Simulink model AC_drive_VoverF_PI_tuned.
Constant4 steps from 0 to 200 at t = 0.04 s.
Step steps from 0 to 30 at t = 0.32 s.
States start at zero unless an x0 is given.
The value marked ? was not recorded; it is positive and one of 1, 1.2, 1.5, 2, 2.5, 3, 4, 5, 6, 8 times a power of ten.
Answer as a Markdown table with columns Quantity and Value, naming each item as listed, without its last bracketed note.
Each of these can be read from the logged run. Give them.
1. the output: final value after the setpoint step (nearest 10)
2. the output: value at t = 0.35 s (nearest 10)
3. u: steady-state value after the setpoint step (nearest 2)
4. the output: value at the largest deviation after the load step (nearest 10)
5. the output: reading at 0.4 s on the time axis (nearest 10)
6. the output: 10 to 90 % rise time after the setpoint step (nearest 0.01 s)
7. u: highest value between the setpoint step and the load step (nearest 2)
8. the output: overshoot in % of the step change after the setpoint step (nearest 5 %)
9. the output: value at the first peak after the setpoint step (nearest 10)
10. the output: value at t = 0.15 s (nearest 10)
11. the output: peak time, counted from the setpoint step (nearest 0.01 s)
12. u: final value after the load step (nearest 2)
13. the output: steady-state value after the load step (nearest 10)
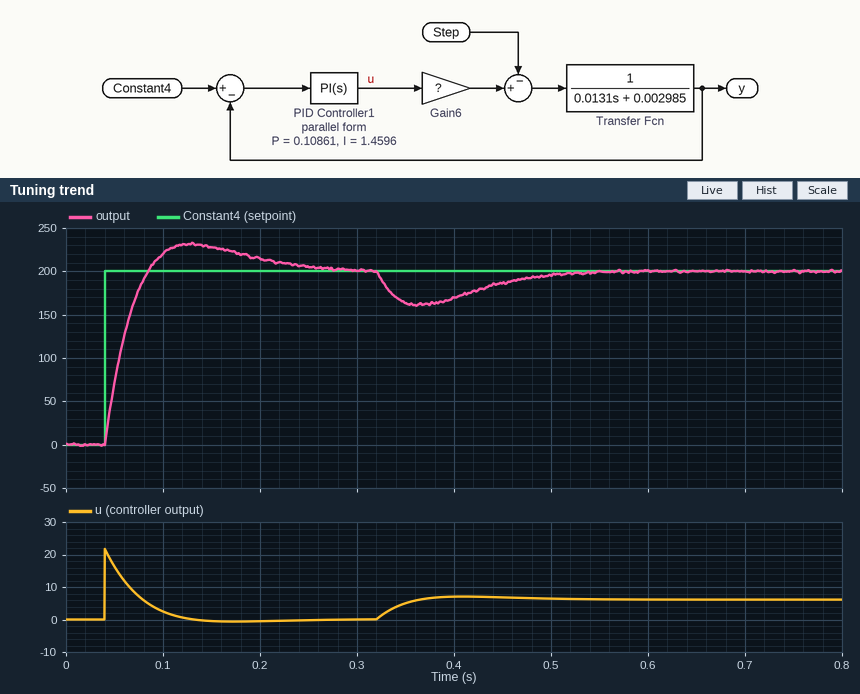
| Quantity | Value |
|---|---|
| the output: final value after the setpoint step | 200 |
| the output: value at t = 0.35 s | 160 |
| u: steady-state value after the setpoint step | 0 |
| the output: value at the largest deviation after the load step | 160 |
| the output: reading at 0.4 s on the time axis | 170 |
| the output: 10 to 90 % rise time after the setpoint step | 0.03 s |
| u: highest value between the setpoint step and the load step | 22 |
| the output: overshoot in % of the step change after the setpoint step | 15 % |
| the output: value at the first peak after the setpoint step | 230 |
| the output: value at t = 0.15 s | 230 |
| the output: peak time, counted from the setpoint step | 0.09 s |
| u: final value after the load step | 6 |
| the output: steady-state value after the load step | 200 |
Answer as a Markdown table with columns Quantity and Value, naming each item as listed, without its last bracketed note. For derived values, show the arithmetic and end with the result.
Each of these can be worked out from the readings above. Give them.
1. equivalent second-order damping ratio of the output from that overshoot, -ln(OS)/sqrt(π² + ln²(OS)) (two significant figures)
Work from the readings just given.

| Quantity | Value |
|---|---|
| equivalent second-order damping ratio of the output from that overshoot, -ln(OS)/sqrt(π² + ln²(OS)) | ln(0.15) = -1.897; 1.897 / sqrt(9.870 + 3.599) = 0.52 |
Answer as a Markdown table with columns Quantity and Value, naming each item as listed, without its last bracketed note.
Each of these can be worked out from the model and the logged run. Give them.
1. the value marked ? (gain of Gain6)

| Quantity | Value |
|---|---|
| the value marked ? | 5 |
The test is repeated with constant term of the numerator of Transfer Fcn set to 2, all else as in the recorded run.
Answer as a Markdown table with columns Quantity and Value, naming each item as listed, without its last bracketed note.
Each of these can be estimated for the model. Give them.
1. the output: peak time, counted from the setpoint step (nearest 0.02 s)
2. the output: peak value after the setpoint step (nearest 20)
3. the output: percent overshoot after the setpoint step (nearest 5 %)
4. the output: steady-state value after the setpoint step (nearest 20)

| Quantity | Value |
|---|---|
| the output: peak time, counted from the setpoint step | 0.06 s |
| the output: peak value after the setpoint step | 220 |
| the output: percent overshoot after the setpoint step | 10 % |
| the output: steady-state value after the setpoint step | 200 |
